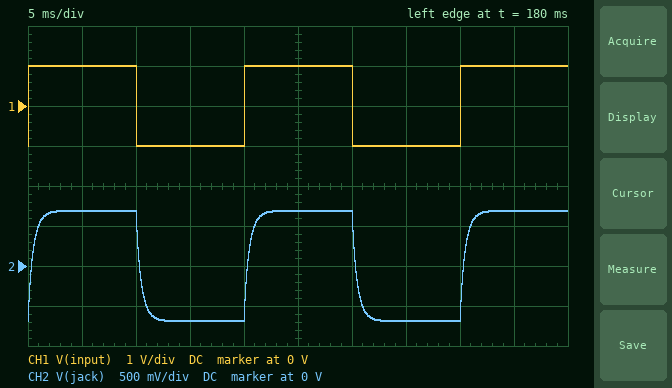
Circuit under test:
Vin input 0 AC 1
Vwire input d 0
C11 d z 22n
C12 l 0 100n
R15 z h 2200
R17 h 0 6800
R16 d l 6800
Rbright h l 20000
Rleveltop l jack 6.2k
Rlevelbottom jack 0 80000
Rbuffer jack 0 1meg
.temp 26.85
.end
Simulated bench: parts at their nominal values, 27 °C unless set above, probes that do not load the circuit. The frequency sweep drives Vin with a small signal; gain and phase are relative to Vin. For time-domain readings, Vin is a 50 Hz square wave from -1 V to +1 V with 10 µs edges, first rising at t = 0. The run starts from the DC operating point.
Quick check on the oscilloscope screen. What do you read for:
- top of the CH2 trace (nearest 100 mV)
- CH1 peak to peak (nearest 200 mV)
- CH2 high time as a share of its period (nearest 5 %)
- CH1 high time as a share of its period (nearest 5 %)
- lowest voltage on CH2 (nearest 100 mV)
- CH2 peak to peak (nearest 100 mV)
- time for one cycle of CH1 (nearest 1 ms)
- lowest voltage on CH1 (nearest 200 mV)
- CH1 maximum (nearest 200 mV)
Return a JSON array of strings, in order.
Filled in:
["700 mV", "2.0 V", "50 %", "50 %", "-700 mV", "1.4 V", "20 ms", "-1.0 V", "1.0 V"]
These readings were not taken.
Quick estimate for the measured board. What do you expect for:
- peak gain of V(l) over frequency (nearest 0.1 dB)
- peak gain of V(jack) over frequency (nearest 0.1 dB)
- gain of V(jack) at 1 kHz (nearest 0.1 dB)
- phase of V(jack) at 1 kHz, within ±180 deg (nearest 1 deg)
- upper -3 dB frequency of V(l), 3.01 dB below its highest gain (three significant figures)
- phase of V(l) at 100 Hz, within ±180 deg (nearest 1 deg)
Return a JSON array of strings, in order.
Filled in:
["-2.5 dB", "-3.2 dB", "-12.8 dB", "-66 deg", "323 Hz", "-17 deg"]
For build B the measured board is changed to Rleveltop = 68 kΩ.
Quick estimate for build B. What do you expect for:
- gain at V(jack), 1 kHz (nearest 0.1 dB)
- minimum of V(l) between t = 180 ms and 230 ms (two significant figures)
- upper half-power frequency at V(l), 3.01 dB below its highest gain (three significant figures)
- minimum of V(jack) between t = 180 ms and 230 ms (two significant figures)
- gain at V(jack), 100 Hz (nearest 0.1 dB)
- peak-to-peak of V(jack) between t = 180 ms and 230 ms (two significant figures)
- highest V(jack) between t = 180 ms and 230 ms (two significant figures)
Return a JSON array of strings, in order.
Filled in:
["-17.7 dB", "-770 mV", "314 Hz", "-400 mV", "-8.4 dB", "800 mV", "400 mV"]
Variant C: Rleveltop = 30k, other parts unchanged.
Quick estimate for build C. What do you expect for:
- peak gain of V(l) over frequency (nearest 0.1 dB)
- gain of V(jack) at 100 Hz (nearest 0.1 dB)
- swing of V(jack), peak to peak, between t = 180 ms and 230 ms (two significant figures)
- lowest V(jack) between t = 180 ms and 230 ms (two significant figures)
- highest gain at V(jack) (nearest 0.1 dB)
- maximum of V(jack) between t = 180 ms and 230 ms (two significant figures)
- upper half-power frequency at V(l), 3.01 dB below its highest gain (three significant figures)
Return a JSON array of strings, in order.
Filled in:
["-2.4 dB", "-5.8 dB", "1.1 V", "-540 mV", "-5.4 dB", "540 mV", "318 Hz"]
